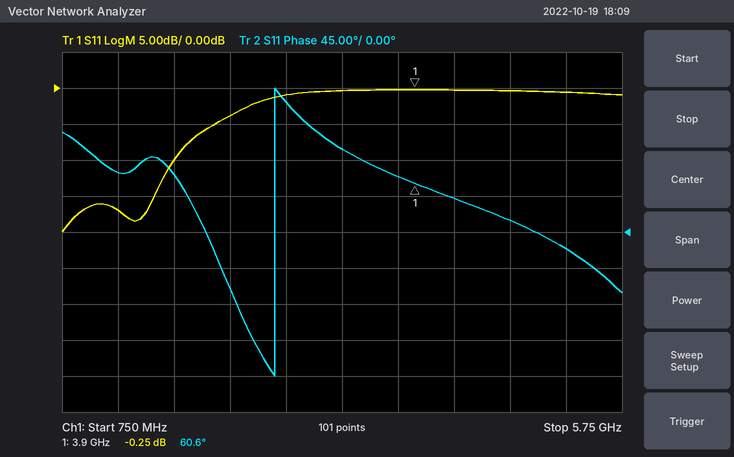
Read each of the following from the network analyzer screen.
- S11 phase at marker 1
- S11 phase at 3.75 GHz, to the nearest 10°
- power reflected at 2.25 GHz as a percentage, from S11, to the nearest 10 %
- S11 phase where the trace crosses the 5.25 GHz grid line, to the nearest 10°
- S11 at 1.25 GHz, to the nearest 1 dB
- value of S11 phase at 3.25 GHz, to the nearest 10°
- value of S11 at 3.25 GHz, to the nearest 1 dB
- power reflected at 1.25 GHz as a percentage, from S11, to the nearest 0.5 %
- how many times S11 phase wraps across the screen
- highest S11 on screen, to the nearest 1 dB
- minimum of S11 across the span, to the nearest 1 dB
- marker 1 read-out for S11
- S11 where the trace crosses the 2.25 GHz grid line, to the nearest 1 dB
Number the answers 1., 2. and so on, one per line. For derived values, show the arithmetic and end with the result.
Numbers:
1. 60.6°
2. 70°
3. 10^(-4/10) ≈ 40 %
4. -20°
5. -17 dB
6. 100°
7. 0 dB
8. 10^(-17/10) ≈ 2.0 %
9. 1
10. 0 dB
11. -20 dB
12. -0.25 dB
13. -4 dB
